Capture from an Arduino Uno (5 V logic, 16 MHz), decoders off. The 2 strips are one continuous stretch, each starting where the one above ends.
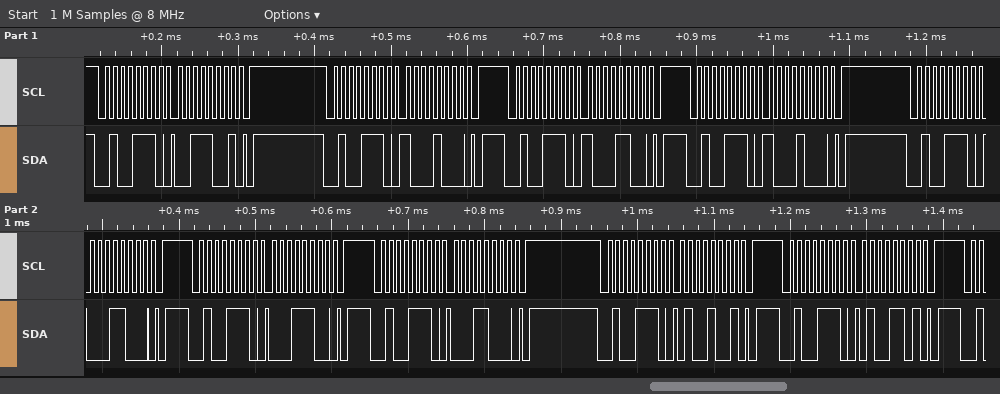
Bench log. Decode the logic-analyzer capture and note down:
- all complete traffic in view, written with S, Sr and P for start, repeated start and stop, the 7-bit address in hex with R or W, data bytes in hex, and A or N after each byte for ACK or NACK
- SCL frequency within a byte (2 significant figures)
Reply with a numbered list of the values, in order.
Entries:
1. S 27W A 39 A P S 27W A 88 A P S 27W A 8C A P S 27W A 88 A P S 27W A 18 A P S 27W A 1C A P S 27W A 18 A P S 27W A 49 A P S 27W A 4D A P
2. 100 kHz
